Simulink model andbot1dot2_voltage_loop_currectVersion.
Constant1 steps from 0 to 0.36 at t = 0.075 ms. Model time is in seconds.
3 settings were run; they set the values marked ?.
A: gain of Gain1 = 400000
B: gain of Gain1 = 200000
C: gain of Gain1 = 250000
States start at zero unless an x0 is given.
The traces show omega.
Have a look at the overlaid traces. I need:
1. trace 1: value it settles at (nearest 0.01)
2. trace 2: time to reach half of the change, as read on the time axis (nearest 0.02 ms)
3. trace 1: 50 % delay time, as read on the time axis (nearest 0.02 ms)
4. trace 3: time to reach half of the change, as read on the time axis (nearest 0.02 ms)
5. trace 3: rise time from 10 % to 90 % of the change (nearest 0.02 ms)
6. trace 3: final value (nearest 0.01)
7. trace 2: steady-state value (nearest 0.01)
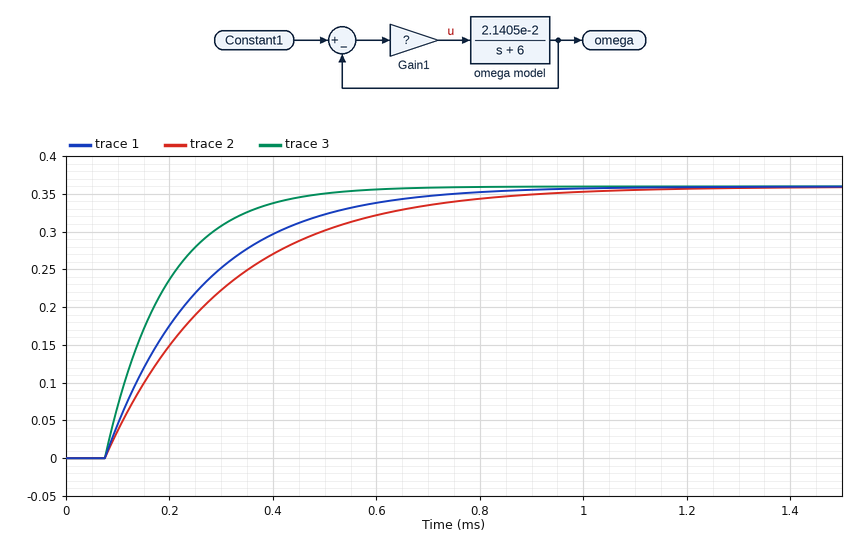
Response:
0.36
0.24 ms
0.20 ms
0.16 ms
0.26 ms
0.36
0.36
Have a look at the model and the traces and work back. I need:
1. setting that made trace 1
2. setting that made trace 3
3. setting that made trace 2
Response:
C
A
B
